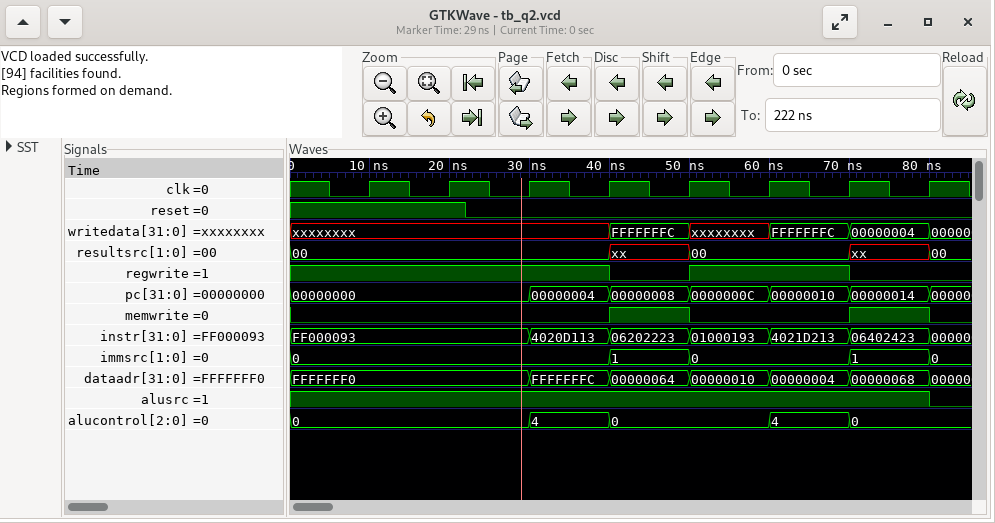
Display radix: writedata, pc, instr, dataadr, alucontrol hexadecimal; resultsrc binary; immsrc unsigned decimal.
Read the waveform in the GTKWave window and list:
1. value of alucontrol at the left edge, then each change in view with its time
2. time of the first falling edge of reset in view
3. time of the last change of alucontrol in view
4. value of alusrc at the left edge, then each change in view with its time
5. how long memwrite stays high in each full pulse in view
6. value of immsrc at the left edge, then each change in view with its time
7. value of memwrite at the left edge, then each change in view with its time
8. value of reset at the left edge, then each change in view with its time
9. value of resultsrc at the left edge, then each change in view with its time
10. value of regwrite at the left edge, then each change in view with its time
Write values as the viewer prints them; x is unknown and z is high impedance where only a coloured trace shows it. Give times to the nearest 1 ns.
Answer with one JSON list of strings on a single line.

["0, 4 at 30 ns, 0 at 40 ns, 4 at 60 ns, 0 at 70 ns", "22 ns", "70 ns", "1, 0 at 80 ns", "10 ns, 10 ns", "0, 1 at 40 ns, 0 at 50 ns, 1 at 70 ns, 0 at 80 ns", "0, 1 at 40 ns, 0 at 50 ns, 1 at 70 ns, 0 at 80 ns", "1, 0 at 22 ns", "00, xx at 40 ns, 00 at 50 ns, xx at 70 ns, 00 at 80 ns", "1, 0 at 40 ns, 1 at 50 ns, 0 at 70 ns"]
